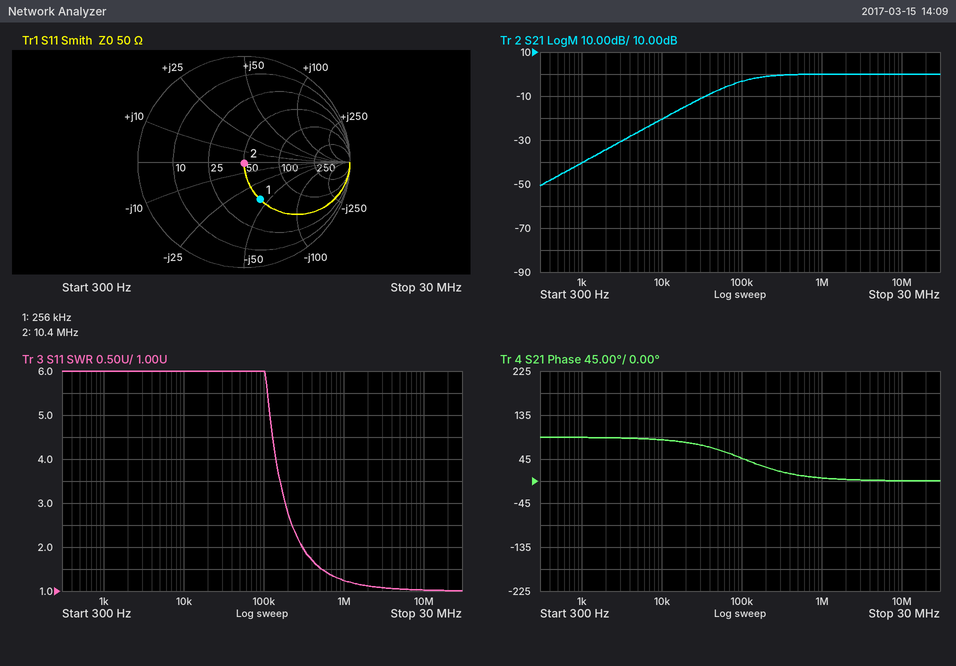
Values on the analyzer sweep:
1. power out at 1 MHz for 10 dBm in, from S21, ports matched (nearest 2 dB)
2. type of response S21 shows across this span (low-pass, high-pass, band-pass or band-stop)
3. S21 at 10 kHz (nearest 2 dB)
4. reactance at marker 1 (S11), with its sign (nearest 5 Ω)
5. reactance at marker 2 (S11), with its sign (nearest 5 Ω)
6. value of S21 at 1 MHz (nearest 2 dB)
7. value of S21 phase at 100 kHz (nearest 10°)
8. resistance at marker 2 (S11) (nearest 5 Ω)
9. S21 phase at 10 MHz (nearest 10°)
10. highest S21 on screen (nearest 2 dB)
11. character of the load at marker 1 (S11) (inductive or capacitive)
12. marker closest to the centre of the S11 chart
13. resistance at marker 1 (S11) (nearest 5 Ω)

10 dBm
high-pass
-20 dB
-40 Ω
0 Ω
0 dB
50°
50 Ω
0°
0 dB
capacitive
marker 2
50 Ω
